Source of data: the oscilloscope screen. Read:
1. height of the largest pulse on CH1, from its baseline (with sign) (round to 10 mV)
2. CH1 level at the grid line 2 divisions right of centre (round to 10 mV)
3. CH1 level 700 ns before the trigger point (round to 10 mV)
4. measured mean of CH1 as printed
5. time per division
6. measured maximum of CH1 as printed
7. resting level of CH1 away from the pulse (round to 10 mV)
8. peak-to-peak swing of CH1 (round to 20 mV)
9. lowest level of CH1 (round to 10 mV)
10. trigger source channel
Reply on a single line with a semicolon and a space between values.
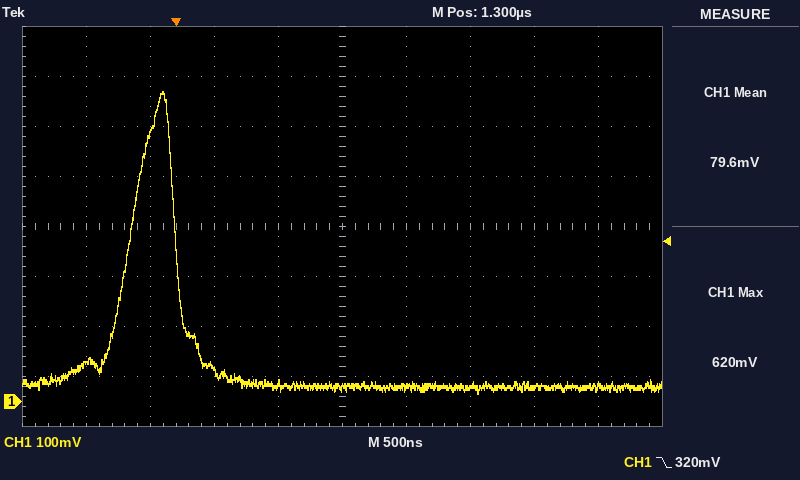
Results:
+590 mV; 30 mV; 80 mV; 79.6 mV; 500 ns; 620 mV; 30 mV; 600 mV; 20 mV; CH1
